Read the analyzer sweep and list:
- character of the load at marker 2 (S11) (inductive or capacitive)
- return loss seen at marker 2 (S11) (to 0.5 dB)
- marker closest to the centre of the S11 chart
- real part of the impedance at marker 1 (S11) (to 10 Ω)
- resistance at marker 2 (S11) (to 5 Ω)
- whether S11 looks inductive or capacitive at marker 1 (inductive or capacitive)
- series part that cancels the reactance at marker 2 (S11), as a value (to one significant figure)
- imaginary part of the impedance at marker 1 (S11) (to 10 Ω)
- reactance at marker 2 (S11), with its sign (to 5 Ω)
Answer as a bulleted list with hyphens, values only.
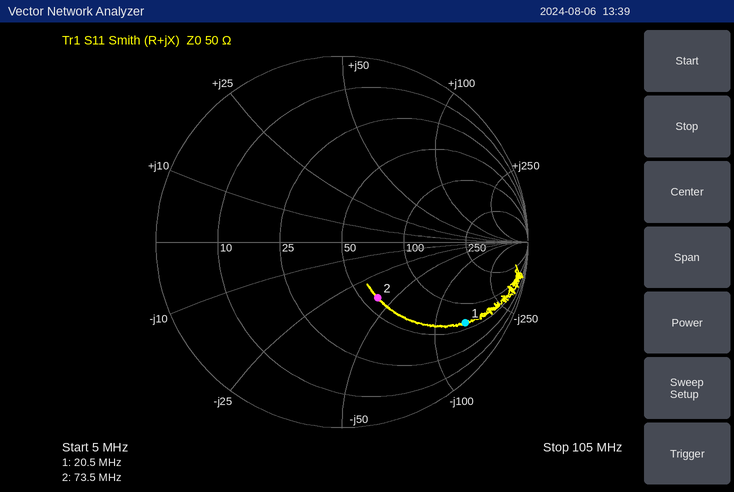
- capacitive
- 9.0 dB
- marker 2
- 60 Ω
- 60 Ω
- capacitive
- 90 nH
- -140 Ω
- -40 Ω
